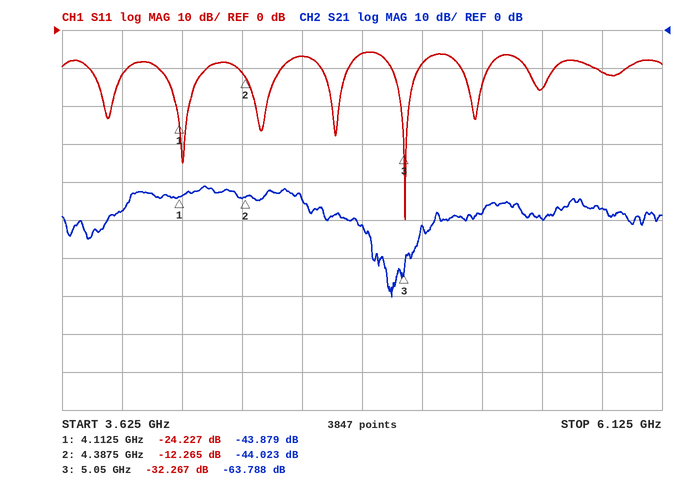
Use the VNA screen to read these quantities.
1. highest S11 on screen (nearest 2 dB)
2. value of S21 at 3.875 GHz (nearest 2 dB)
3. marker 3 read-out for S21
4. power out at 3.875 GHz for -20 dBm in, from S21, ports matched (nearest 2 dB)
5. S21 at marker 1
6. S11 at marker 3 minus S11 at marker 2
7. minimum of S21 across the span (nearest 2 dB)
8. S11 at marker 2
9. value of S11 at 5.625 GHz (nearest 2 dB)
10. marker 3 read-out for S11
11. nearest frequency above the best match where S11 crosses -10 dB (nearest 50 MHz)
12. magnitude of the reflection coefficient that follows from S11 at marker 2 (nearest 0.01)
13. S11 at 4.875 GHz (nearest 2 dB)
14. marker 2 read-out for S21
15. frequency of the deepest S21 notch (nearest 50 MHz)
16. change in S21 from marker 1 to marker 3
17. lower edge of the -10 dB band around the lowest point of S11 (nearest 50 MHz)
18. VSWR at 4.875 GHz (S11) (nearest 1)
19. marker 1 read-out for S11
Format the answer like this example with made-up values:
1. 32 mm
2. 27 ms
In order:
1. -6 dB
2. -48 dB
3. -63.788 dB
4. -68 dBm
5. -43.879 dB
6. -20.002 dB
7. -70 dB
8. -12.265 dB
9. -16 dB
10. -32.267 dB
11. 5.10 GHz
12. 0.24
13. -6 dB
14. -44.023 dB
15. 5.00 GHz
16. -19.909 dB
17. 5.00 GHz
18. 3
19. -24.227 dB
